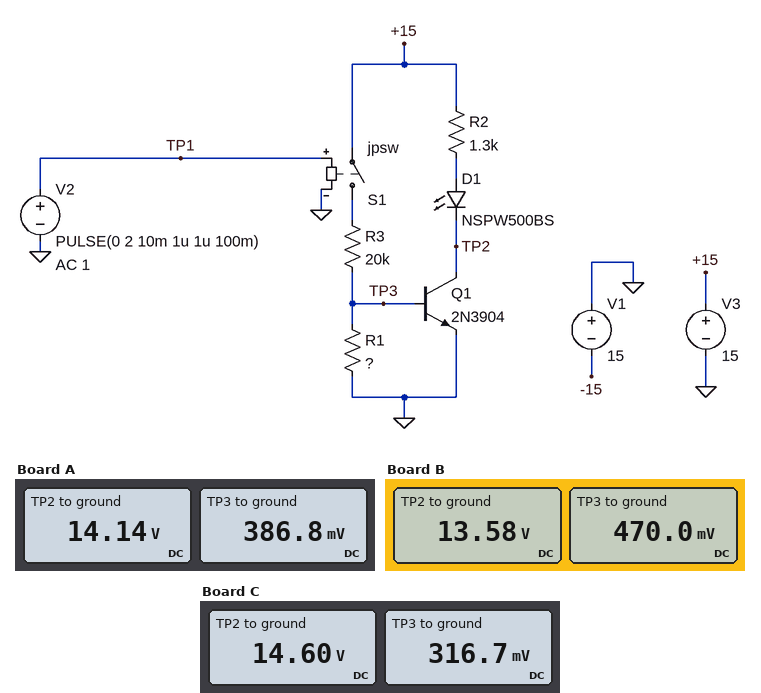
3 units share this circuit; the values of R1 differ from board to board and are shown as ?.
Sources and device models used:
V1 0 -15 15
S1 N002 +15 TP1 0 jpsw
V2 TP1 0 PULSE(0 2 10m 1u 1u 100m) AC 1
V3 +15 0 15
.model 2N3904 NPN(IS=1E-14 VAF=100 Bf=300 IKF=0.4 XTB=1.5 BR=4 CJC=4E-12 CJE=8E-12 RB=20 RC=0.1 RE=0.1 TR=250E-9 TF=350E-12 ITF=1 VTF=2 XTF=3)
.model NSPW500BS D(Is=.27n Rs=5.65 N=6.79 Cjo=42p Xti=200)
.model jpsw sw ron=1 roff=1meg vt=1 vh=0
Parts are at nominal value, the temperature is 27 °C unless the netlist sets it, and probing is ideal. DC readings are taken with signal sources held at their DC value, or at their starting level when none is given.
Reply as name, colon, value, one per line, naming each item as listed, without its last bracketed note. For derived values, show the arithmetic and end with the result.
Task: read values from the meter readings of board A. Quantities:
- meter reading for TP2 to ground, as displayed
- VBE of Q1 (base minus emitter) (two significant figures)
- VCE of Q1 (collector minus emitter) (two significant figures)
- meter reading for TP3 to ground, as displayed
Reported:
meter reading for TP2 to ground, as displayed: 14.14 V
VBE of Q1 (base minus emitter): 386.8 mV = 390 mV
VCE of Q1 (collector minus emitter): 14.14 V = 14 V
meter reading for TP3 to ground, as displayed: 386.8 mV
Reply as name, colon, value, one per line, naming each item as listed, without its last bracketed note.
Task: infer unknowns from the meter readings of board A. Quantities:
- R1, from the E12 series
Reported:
R1, from the E12 series: 27 kΩ
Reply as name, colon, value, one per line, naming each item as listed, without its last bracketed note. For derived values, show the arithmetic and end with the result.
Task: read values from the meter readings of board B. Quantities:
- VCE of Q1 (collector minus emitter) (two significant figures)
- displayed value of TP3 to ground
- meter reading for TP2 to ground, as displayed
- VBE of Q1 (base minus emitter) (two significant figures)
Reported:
VCE of Q1 (collector minus emitter): 13.58 V = 14 V
displayed value of TP3 to ground: 470.0 mV
meter reading for TP2 to ground, as displayed: 13.58 V
VBE of Q1 (base minus emitter): 470 mV = 470 mV
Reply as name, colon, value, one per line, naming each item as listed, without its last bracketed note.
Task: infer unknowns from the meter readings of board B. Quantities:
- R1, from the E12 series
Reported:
R1, from the E12 series: 33 kΩ
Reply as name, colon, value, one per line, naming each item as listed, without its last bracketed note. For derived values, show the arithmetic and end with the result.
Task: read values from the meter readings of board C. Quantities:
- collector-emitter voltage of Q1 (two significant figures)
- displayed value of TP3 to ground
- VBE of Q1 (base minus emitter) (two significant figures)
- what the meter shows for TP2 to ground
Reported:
collector-emitter voltage of Q1: 14.6 V = 15 V
displayed value of TP3 to ground: 316.7 mV
VBE of Q1 (base minus emitter): 316.7 mV = 320 mV
what the meter shows for TP2 to ground: 14.60 V
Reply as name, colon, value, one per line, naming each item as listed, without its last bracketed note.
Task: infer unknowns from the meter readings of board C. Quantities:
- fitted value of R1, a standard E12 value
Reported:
fitted value of R1, a standard E12 value: 22 kΩ
